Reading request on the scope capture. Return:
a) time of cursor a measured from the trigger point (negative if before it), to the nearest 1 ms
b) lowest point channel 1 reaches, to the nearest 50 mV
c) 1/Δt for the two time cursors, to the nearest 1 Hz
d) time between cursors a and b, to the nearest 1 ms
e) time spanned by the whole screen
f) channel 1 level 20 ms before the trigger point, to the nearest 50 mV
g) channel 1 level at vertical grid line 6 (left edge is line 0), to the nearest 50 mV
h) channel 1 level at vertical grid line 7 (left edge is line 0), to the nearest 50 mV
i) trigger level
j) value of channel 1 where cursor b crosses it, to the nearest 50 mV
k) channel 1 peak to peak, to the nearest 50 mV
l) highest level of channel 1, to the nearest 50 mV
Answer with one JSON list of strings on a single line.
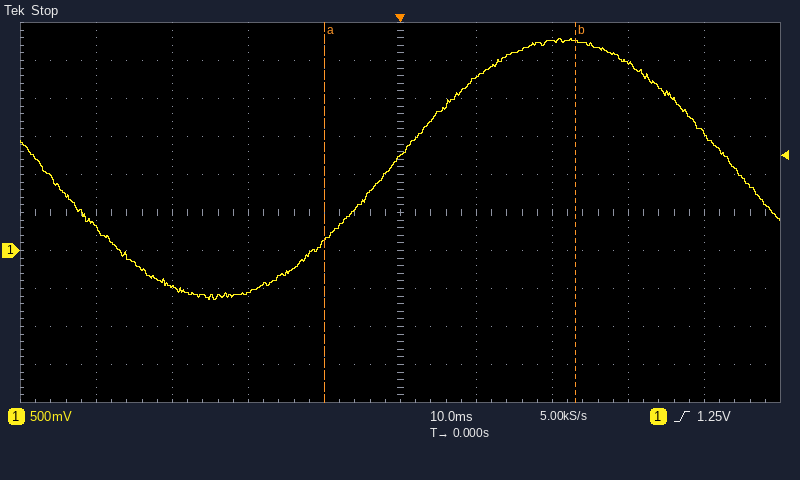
["-10 ms", "-650 mV", "30 Hz", "33 ms", "100 ms", "-550 mV", "2.30 V", "2.75 V", "1.25 V", "2.75 V", "3.45 V", "2.80 V"]
